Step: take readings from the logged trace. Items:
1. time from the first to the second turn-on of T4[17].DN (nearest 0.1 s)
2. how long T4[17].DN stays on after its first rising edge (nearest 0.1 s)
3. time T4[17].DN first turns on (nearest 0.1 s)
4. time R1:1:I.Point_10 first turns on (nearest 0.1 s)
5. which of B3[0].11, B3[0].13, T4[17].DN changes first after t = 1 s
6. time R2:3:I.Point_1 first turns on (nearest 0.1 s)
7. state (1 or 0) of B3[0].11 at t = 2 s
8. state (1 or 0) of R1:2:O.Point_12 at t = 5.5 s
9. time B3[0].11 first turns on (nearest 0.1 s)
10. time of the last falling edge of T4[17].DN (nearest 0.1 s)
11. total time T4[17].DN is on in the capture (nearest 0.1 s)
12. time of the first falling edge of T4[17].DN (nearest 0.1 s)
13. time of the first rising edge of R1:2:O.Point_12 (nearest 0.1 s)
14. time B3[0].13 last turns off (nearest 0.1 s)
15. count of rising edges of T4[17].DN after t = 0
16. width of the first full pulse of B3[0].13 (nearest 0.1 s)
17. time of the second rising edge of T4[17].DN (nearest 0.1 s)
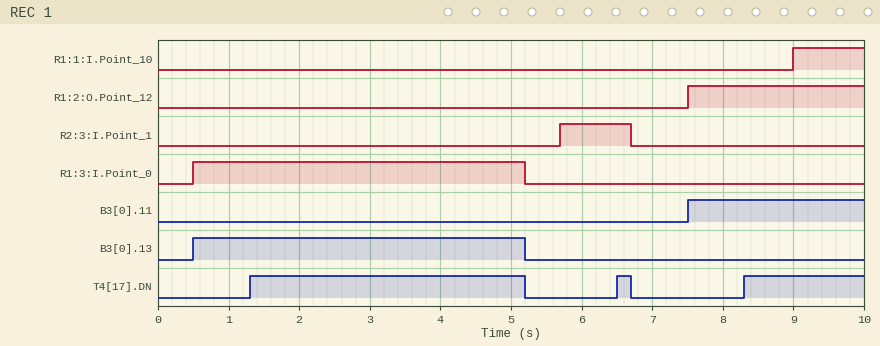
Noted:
5.2 s
3.9 s
1.3 s
9.0 s
T4[17].DN
5.7 s
0
0
7.5 s
6.7 s
5.8 s
5.2 s
7.5 s
5.2 s
3
4.7 s
6.5 s
